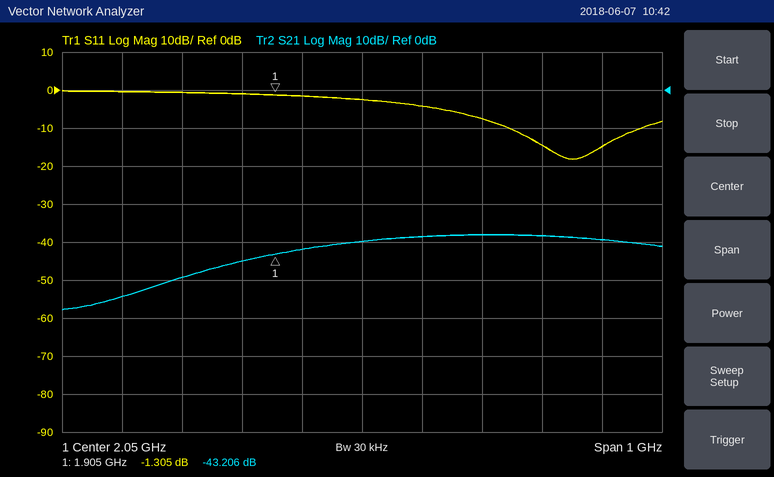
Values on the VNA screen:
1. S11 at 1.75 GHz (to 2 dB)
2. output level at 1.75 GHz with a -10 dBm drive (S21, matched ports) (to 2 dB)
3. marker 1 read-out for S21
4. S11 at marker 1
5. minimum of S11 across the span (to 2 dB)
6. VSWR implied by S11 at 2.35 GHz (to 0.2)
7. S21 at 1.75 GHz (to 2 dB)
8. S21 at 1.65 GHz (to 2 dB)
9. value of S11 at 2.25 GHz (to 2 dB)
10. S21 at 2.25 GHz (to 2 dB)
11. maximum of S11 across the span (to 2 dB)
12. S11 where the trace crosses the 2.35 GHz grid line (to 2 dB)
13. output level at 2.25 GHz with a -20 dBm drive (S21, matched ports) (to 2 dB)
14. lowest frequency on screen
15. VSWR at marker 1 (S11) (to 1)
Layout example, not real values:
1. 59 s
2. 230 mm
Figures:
1. 0 dB
2. -60 dBm
3. -43.206 dB
4. -1.305 dB
5. -18 dB
6. 1.4
7. -50 dB
8. -54 dB
9. -8 dB
10. -38 dB
11. 0 dB
12. -14 dB
13. -58 dBm
14. 1.55 GHz
15. 13
